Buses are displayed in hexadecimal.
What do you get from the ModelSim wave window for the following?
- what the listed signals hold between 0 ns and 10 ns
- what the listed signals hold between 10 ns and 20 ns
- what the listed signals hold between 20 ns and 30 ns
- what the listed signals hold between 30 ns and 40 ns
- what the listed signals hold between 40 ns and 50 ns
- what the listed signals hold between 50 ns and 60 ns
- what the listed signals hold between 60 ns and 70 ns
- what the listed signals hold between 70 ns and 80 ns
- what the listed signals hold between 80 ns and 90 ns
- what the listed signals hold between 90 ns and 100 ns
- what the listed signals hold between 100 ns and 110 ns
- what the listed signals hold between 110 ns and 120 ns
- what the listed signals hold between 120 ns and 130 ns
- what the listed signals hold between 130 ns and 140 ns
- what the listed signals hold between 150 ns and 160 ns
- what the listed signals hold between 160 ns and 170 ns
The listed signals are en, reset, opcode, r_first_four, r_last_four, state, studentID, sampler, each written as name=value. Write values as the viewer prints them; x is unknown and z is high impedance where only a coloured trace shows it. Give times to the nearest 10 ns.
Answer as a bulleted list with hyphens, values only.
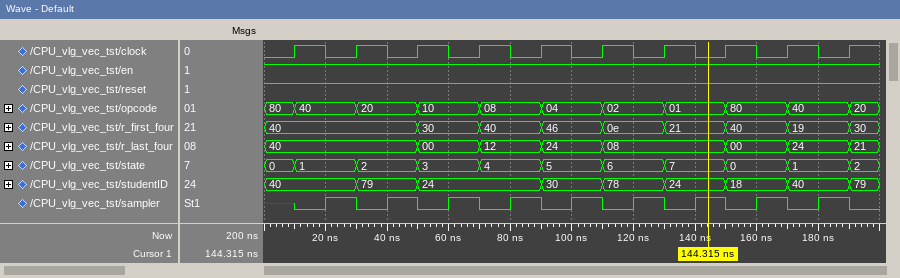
- en=1, reset=1, opcode=80, r_first_four=40, r_last_four=40, state=0, studentID=40, sampler=x
- en=1, reset=1, opcode=40, r_first_four=40, r_last_four=40, state=1, studentID=40, sampler=0
- en=1, reset=1, opcode=40, r_first_four=40, r_last_four=40, state=1, studentID=40, sampler=1
- en=1, reset=1, opcode=20, r_first_four=40, r_last_four=40, state=2, studentID=79, sampler=0
- en=1, reset=1, opcode=20, r_first_four=40, r_last_four=40, state=2, studentID=79, sampler=1
- en=1, reset=1, opcode=10, r_first_four=30, r_last_four=00, state=3, studentID=24, sampler=0
- en=1, reset=1, opcode=10, r_first_four=30, r_last_four=00, state=3, studentID=24, sampler=1
- en=1, reset=1, opcode=08, r_first_four=40, r_last_four=12, state=4, studentID=24, sampler=0
- en=1, reset=1, opcode=08, r_first_four=40, r_last_four=12, state=4, studentID=24, sampler=1
- en=1, reset=1, opcode=04, r_first_four=46, r_last_four=24, state=5, studentID=30, sampler=0
- en=1, reset=1, opcode=04, r_first_four=46, r_last_four=24, state=5, studentID=30, sampler=1
- en=1, reset=1, opcode=02, r_first_four=0e, r_last_four=08, state=6, studentID=78, sampler=0
- en=1, reset=1, opcode=02, r_first_four=0e, r_last_four=08, state=6, studentID=78, sampler=1
- en=1, reset=1, opcode=01, r_first_four=21, r_last_four=08, state=7, studentID=24, sampler=0
- en=1, reset=1, opcode=80, r_first_four=40, r_last_four=00, state=0, studentID=18, sampler=0
- en=1, reset=1, opcode=80, r_first_four=40, r_last_four=00, state=0, studentID=18, sampler=1
